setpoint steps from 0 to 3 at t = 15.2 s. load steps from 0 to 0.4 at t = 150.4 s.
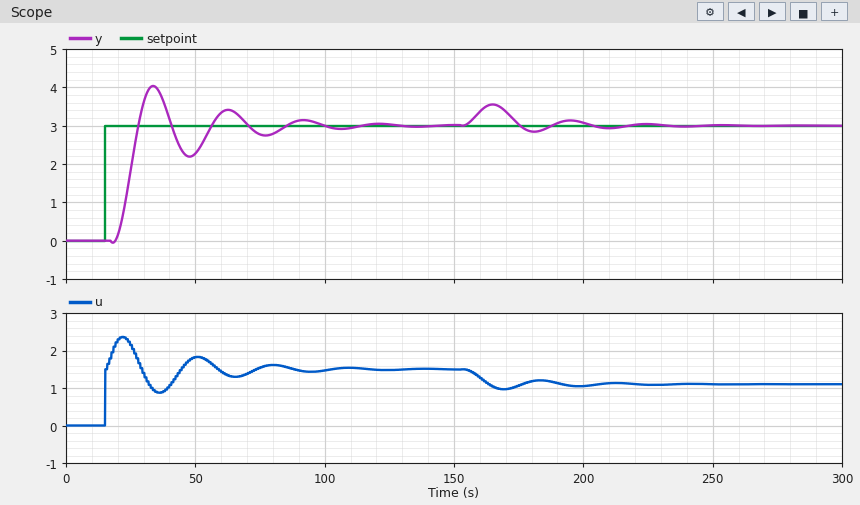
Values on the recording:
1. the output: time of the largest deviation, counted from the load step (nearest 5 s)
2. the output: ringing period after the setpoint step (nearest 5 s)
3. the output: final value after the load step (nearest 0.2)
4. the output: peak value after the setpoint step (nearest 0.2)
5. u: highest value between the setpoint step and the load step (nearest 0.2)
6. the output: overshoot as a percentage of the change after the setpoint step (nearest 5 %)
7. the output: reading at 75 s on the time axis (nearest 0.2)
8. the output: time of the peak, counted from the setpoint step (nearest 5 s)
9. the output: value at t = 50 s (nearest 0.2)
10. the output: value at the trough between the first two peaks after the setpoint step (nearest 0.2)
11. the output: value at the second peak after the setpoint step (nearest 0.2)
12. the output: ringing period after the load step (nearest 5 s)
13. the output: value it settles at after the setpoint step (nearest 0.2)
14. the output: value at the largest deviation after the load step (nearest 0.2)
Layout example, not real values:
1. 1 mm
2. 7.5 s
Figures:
1. 15 s
2. 30 s
3. 3.0
4. 4.0
5. 2.4
6. 35 %
7. 2.8
8. 20 s
9. 2.2
10. 2.2
11. 3.4
12. 30 s
13. 3.0
14. 3.6
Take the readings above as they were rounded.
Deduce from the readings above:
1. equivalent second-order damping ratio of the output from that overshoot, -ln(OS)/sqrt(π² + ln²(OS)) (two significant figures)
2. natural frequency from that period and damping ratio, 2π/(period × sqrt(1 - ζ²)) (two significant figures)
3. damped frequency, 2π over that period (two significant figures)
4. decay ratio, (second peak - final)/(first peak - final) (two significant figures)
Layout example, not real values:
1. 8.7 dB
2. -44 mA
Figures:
1. 0.32
2. 0.22 rad/s
3. 0.21 rad/s
4. 0.40
